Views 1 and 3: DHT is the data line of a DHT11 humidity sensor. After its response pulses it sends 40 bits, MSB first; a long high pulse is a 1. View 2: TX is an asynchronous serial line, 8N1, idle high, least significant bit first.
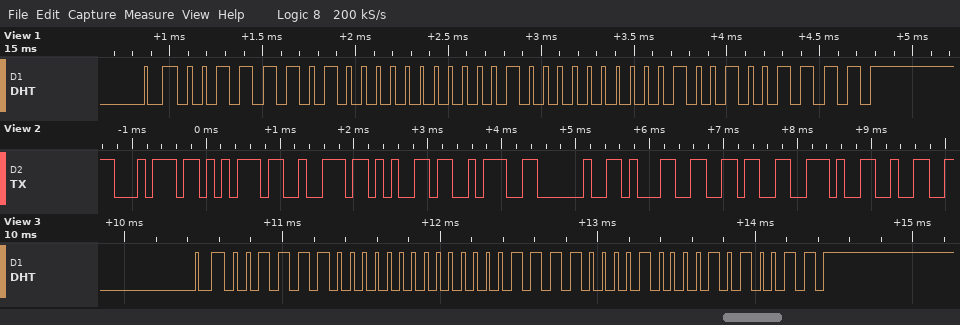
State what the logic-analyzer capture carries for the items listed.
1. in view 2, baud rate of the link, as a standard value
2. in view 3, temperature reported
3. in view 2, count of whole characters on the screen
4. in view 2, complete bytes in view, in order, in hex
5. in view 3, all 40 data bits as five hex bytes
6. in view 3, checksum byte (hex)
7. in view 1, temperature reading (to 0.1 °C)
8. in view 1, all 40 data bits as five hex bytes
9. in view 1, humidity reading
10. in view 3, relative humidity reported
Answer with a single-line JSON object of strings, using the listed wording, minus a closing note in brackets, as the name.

{"in view 2, baud rate of the link, as a standard value": "9600 baud", "in view 3, temperature reported": "15.8 °C", "in view 2, count of whole characters on the screen": "10", "in view 2, complete bytes in view, in order, in hex": "74 75 72 65 3A 20 31 36 2E 32", "in view 3, all 40 data bits as five hex bytes": "3C 00 0F 08 53", "in view 3, checksum byte": "0x53", "in view 1, temperature reading": "16.2 °C", "in view 1, all 40 data bits as five hex bytes": "3D 00 10 02 4F", "in view 1, humidity reading": "61 %", "in view 3, relative humidity reported": "60 %"}
